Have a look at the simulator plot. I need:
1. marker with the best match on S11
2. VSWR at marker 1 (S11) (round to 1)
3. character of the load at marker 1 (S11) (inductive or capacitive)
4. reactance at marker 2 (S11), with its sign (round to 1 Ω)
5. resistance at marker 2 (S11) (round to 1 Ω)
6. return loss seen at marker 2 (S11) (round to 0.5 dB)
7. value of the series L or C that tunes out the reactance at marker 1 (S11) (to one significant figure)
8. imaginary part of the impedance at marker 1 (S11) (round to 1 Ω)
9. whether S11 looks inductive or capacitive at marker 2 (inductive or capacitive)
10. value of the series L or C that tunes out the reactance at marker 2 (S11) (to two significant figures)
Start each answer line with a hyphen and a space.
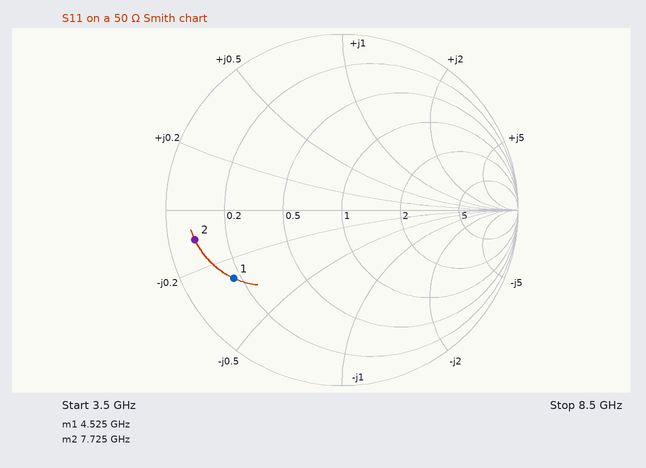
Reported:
- marker 1
- 6
- capacitive
- -5 Ω
- 4 Ω
- 1.5 dB
- 500 pH
- -14 Ω
- capacitive
- 100 pH
